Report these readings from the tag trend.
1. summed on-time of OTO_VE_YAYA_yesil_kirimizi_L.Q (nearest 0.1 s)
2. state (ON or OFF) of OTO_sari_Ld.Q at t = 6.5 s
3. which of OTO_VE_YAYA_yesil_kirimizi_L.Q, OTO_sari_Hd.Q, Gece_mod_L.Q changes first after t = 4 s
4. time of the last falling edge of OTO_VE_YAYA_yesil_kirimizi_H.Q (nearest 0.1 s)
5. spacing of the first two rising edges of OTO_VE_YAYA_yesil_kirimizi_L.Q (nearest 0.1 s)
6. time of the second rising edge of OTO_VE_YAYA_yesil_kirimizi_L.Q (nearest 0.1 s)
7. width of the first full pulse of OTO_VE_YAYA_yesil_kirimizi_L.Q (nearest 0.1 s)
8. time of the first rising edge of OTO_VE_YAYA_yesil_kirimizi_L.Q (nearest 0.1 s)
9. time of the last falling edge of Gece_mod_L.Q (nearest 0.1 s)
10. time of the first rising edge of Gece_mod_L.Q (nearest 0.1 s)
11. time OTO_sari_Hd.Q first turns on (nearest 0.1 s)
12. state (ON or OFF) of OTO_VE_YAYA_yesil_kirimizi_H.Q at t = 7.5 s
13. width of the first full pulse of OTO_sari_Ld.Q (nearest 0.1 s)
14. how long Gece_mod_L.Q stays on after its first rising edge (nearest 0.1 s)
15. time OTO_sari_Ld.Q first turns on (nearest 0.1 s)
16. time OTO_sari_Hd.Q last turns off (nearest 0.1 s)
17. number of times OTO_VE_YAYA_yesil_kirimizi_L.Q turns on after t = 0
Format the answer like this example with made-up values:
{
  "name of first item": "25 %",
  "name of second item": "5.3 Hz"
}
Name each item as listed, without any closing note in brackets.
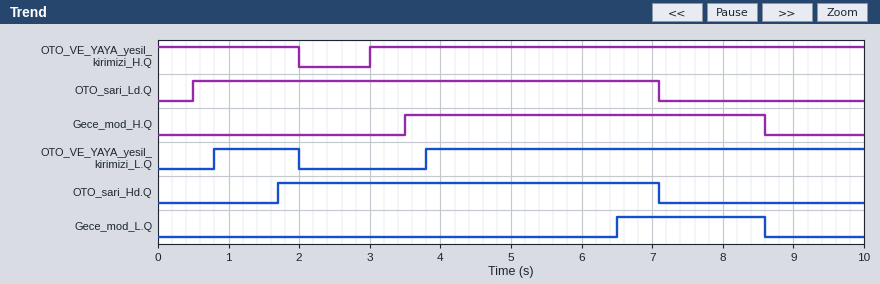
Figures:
{
  "summed on-time of OTO_VE_YAYA_yesil_kirimizi_L.Q": "7.4 s",
  "state (ON or OFF) of OTO_sari_Ld.Q at t = 6.5 s": "ON",
  "which of OTO_VE_YAYA_yesil_kirimizi_L.Q, OTO_sari_Hd.Q, Gece_mod_L.Q changes first after t = 4 s": "Gece_mod_L.Q",
  "time of the last falling edge of OTO_VE_YAYA_yesil_kirimizi_H.Q": "2.0 s",
  "spacing of the first two rising edges of OTO_VE_YAYA_yesil_kirimizi_L.Q": "3.0 s",
  "time of the second rising edge of OTO_VE_YAYA_yesil_kirimizi_L.Q": "3.8 s",
  "width of the first full pulse of OTO_VE_YAYA_yesil_kirimizi_L.Q": "1.2 s",
  "time of the first rising edge of OTO_VE_YAYA_yesil_kirimizi_L.Q": "0.8 s",
  "time of the last falling edge of Gece_mod_L.Q": "8.6 s",
  "time of the first rising edge of Gece_mod_L.Q": "6.5 s",
  "time OTO_sari_Hd.Q first turns on": "1.7 s",
  "state (ON or OFF) of OTO_VE_YAYA_yesil_kirimizi_H.Q at t = 7.5 s": "ON",
  "width of the first full pulse of OTO_sari_Ld.Q": "6.6 s",
  "how long Gece_mod_L.Q stays on after its first rising edge": "2.1 s",
  "time OTO_sari_Ld.Q first turns on": "0.5 s",
  "time OTO_sari_Hd.Q last turns off": "7.1 s",
  "number of times OTO_VE_YAYA_yesil_kirimizi_L.Q turns on after t = 0": "2"
}
